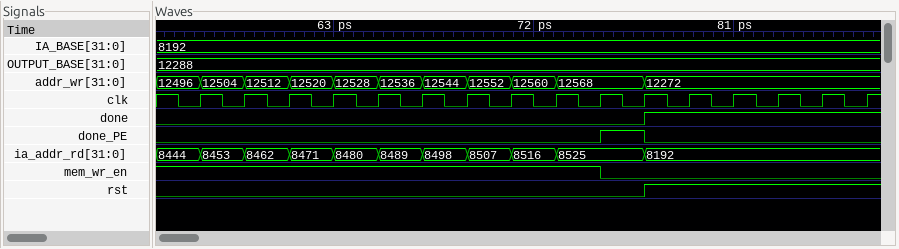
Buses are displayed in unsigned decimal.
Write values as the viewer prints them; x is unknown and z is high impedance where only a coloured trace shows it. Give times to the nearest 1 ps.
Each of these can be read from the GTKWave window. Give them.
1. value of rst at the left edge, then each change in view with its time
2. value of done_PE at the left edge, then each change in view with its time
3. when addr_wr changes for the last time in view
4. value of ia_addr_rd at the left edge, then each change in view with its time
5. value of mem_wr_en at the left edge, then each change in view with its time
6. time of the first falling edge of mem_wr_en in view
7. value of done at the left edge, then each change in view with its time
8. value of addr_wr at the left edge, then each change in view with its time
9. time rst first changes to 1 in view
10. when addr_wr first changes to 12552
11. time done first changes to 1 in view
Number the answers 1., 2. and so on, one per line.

1. 0, 1 at 77 ps
2. 0, 1 at 75 ps, 0 at 77 ps
3. 77 ps
4. 8444, 8453 at 57 ps, 8462 at 59 ps, 8471 at 61 ps, 8480 at 63 ps, 8489 at 65 ps, 8498 at 67 ps, 8507 at 69 ps, 8516 at 71 ps, 8525 at 73 ps, 8192 at 77 ps
5. 1, 0 at 75 ps
6. 75 ps
7. 0, 1 at 77 ps
8. 12496, 12504 at 57 ps, 12512 at 59 ps, 12520 at 61 ps, 12528 at 63 ps, 12536 at 65 ps, 12544 at 67 ps, 12552 at 69 ps, 12560 at 71 ps, 12568 at 73 ps, 12272 at 77 ps
9. 77 ps
10. 69 ps
11. 77 ps
